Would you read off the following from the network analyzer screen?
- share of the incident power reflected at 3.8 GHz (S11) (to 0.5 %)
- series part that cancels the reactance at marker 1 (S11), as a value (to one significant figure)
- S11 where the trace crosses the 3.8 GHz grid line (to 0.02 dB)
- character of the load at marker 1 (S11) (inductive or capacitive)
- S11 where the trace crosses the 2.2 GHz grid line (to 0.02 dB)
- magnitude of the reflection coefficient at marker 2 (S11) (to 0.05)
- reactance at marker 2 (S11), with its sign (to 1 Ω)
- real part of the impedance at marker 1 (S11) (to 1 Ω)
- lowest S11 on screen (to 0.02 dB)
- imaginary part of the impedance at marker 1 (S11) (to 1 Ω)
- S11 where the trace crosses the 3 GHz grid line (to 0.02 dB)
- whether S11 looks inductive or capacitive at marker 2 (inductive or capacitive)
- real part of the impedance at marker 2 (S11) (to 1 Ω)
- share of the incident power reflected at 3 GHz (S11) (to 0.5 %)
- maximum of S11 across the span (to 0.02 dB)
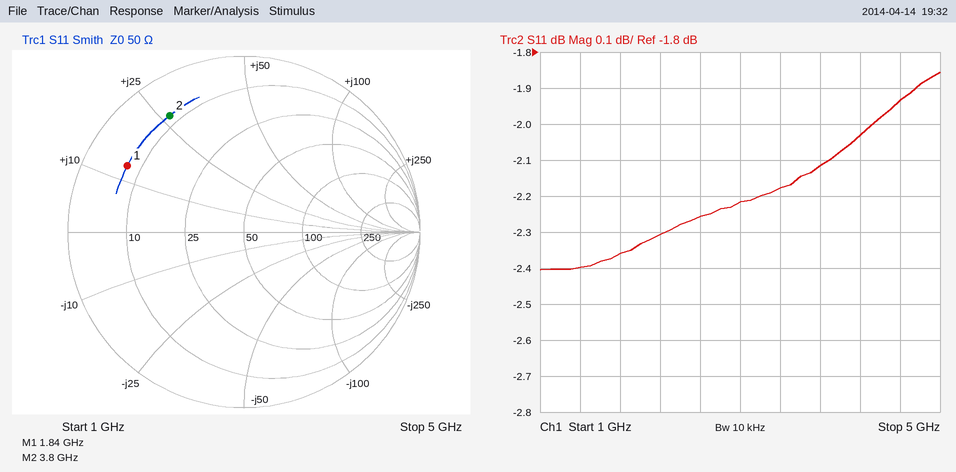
61.5 %
7 pF
-2.12 dB
inductive
-2.30 dB
0.80
+27 Ω
7 Ω
-2.40 dB
+13 Ω
-2.22 dB
inductive
8 Ω
60.0 %
-1.86 dB
